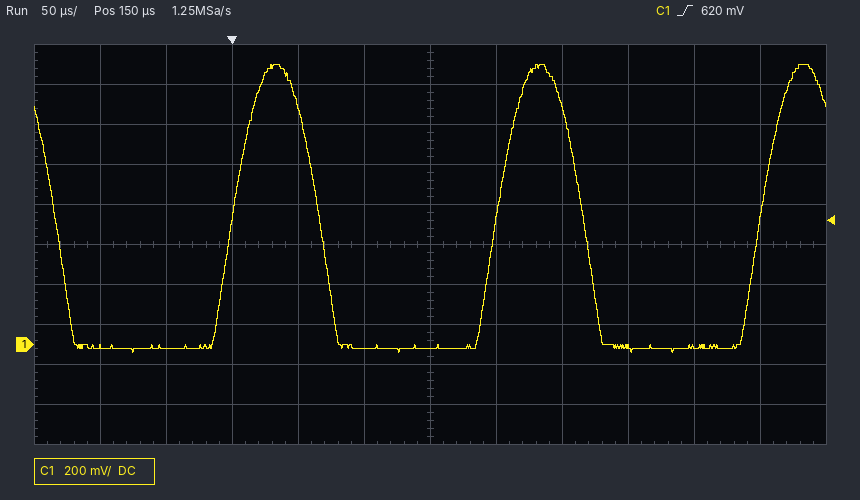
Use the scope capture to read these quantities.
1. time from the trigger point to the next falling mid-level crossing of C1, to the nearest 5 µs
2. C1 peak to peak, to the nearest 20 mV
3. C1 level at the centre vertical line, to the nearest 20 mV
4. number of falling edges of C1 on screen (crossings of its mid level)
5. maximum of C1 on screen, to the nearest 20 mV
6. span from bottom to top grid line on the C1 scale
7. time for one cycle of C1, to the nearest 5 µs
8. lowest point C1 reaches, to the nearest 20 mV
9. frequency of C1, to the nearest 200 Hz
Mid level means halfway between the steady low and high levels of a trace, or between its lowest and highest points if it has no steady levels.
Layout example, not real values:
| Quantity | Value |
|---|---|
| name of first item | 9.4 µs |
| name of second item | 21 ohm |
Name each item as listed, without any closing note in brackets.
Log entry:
| Quantity | Value |
|---|---|
| time from the trigger point to the next falling mid-level crossing of C1, to the nearest 5 µs | 65 µs |
| C1 peak to peak, to the nearest 20 mV | 1.44 V |
| C1 level at the centre vertical line, to the nearest 20 mV | -20 mV |
| number of falling edges of C1 on screen | 3 |
| maximum of C1 on screen, to the nearest 20 mV | 1.40 V |
| span from bottom to top grid line on the C1 scale | 2 V |
| time for one cycle of C1, to the nearest 5 µs | 200 µs |
| lowest point C1 reaches, to the nearest 20 mV | -40 mV |
| frequency of C1, to the nearest 200 Hz | 5.0 kHz |
